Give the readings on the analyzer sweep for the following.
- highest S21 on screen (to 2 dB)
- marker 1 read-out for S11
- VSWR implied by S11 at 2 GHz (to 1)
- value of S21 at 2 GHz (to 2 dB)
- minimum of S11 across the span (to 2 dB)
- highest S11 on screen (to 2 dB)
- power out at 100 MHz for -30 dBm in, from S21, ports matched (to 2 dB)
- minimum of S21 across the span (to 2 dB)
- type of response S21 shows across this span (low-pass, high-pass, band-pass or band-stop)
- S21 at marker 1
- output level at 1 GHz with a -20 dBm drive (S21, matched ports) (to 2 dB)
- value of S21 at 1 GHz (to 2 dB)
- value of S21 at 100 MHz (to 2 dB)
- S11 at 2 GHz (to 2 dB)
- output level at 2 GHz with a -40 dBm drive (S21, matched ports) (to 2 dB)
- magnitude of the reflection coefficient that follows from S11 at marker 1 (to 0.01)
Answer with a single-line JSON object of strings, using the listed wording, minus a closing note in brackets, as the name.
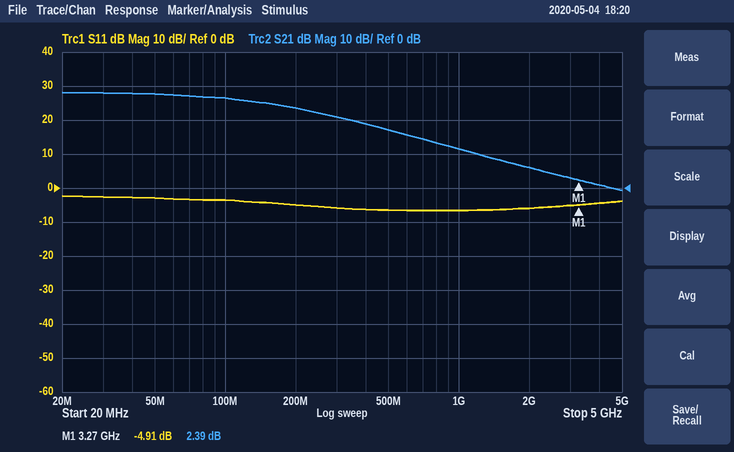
{"highest S21 on screen": "28 dB", "marker 1 read-out for S11": "-4.91 dB", "VSWR implied by S11 at 2 GHz": "3", "value of S21 at 2 GHz": "6 dB", "minimum of S11 across the span": "-6 dB", "highest S11 on screen": "-2 dB", "power out at 100 MHz for -30 dBm in, from S21, ports matched": "-4 dBm", "minimum of S21 across the span": "0 dB", "type of response S21 shows across this span": "low-pass", "S21 at marker 1": "2.39 dB", "output level at 1 GHz with a -20 dBm drive (S21, matched ports)": "-8 dBm", "value of S21 at 1 GHz": "12 dB", "value of S21 at 100 MHz": "26 dB", "S11 at 2 GHz": "-6 dB", "output level at 2 GHz with a -40 dBm drive (S21, matched ports)": "-34 dBm", "magnitude of the reflection coefficient that follows from S11 at marker 1": "0.57"}
